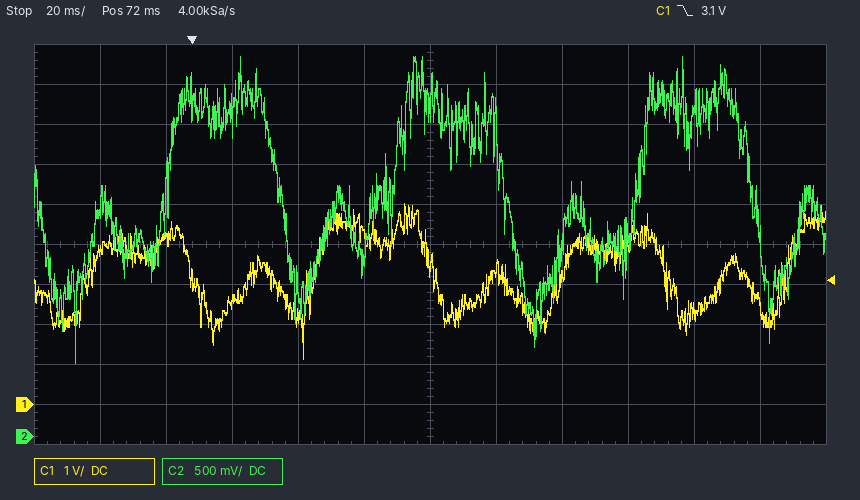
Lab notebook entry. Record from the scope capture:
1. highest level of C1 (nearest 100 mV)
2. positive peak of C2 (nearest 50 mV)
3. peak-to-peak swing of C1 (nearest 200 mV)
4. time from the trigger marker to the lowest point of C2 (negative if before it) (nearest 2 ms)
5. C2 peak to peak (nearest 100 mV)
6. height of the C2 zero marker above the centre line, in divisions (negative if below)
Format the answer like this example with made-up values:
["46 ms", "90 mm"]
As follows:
["5.0 V", "4.75 V", "3.8 V", "-36 ms", "3.80 V", "-4.8 div"]
